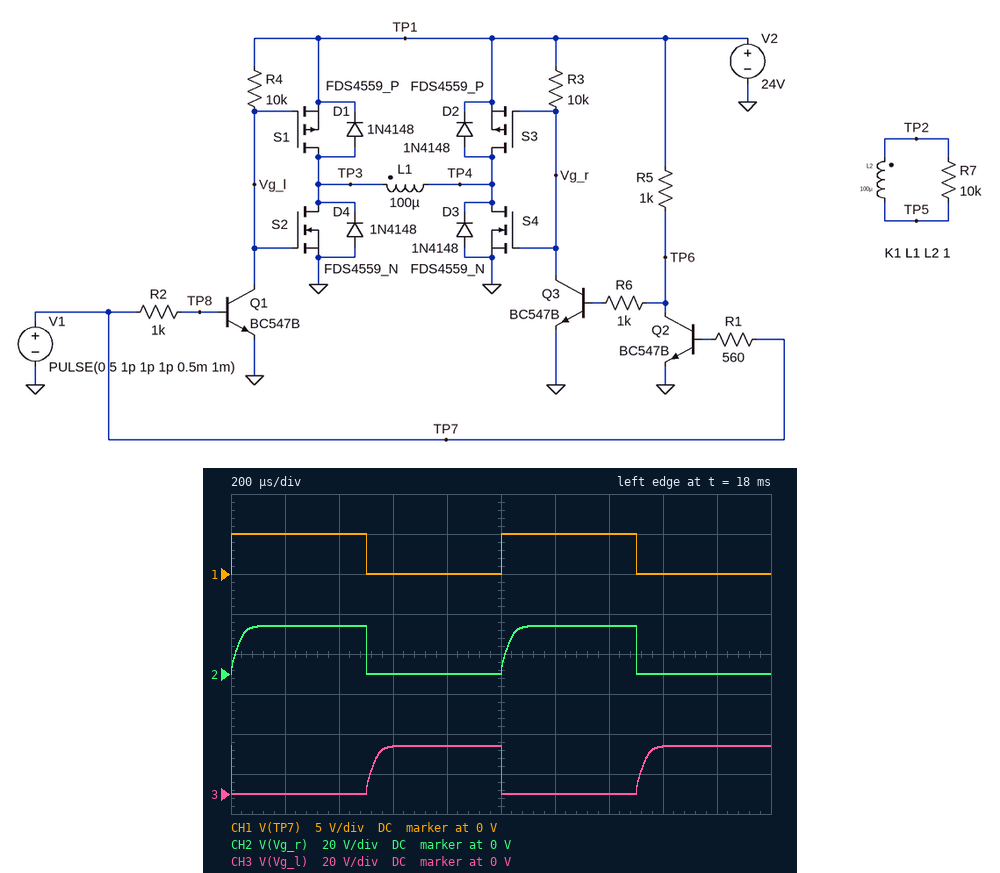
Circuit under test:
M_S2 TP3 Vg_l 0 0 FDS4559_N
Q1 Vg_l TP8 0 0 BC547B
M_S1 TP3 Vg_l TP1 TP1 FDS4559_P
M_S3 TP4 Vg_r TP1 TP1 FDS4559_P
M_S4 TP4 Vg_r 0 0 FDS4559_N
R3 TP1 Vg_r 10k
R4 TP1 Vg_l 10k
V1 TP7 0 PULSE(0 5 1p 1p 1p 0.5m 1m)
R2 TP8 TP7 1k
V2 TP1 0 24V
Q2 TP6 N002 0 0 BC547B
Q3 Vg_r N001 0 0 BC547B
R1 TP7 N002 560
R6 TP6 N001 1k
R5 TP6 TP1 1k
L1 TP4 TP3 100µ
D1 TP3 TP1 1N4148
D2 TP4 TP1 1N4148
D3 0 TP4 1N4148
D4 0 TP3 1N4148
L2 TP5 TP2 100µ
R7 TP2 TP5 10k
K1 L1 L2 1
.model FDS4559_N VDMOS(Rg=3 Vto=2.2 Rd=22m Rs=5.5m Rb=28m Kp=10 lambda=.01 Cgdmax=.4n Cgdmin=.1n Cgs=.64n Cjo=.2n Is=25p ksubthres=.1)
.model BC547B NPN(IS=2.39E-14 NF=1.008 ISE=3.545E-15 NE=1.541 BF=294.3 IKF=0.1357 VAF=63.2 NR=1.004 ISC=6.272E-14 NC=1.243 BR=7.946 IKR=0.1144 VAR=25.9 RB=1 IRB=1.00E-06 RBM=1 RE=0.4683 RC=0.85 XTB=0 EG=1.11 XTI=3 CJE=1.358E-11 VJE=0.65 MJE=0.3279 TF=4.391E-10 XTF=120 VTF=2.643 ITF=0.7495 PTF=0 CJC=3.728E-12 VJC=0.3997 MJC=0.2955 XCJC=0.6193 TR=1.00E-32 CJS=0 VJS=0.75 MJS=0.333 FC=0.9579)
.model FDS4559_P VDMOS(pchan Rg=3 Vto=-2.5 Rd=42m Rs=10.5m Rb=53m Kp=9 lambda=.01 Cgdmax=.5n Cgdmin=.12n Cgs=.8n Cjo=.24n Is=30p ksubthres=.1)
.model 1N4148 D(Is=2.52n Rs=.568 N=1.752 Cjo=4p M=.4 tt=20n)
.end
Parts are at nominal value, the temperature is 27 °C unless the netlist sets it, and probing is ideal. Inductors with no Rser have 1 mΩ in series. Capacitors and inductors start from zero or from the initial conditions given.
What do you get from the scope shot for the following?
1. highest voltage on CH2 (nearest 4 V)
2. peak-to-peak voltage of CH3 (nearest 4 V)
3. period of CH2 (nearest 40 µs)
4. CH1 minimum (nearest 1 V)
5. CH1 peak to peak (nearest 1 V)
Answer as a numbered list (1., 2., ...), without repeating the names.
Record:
1. 24 V
2. 24 V
3. 1.00 ms
4. 0 V
5. 5 V
